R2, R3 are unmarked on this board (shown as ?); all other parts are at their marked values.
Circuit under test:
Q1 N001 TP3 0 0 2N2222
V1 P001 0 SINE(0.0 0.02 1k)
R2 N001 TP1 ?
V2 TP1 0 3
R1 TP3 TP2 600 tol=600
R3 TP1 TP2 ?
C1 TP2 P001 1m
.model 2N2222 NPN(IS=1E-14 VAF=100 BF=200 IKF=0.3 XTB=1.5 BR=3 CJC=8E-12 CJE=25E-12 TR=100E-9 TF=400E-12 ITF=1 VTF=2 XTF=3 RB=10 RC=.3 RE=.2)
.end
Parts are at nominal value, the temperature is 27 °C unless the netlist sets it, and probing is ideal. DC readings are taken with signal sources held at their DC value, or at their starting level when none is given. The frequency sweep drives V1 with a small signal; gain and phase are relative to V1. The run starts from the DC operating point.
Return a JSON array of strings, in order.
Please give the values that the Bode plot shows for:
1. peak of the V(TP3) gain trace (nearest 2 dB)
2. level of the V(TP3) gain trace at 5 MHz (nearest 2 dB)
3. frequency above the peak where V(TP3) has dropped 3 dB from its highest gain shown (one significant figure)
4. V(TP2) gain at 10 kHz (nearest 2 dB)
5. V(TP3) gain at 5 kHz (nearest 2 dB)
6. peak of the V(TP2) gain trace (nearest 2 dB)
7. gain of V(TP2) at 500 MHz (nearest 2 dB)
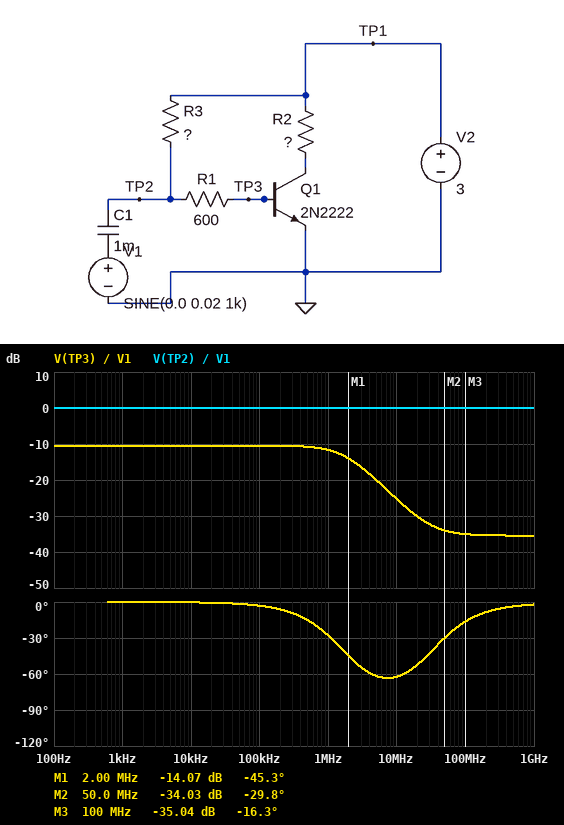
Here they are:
["-10 dB", "-20 dB", "2 MHz", "0 dB", "-10 dB", "0 dB", "0 dB"]
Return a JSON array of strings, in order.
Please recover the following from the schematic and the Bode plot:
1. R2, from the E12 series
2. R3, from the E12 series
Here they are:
["47 Ω", "18 kΩ"]
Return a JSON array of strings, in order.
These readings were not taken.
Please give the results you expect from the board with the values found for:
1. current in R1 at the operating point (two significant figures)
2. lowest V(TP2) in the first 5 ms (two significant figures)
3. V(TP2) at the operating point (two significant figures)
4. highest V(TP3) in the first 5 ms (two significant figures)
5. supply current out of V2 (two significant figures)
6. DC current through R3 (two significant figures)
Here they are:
["120 µA", "800 mV", "820 mV", "750 mV", "23 mA", "120 µA"]
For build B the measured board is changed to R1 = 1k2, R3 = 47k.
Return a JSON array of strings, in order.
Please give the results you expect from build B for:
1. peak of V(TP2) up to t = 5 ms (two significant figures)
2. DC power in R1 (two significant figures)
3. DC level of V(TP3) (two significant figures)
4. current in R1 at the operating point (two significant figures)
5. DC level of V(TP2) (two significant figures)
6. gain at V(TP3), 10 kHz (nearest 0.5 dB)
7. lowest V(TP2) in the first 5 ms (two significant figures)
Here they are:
["790 mV", "2.7 µW", "720 mV", "47 µA", "770 mV", "-9.5 dB", "750 mV"]
